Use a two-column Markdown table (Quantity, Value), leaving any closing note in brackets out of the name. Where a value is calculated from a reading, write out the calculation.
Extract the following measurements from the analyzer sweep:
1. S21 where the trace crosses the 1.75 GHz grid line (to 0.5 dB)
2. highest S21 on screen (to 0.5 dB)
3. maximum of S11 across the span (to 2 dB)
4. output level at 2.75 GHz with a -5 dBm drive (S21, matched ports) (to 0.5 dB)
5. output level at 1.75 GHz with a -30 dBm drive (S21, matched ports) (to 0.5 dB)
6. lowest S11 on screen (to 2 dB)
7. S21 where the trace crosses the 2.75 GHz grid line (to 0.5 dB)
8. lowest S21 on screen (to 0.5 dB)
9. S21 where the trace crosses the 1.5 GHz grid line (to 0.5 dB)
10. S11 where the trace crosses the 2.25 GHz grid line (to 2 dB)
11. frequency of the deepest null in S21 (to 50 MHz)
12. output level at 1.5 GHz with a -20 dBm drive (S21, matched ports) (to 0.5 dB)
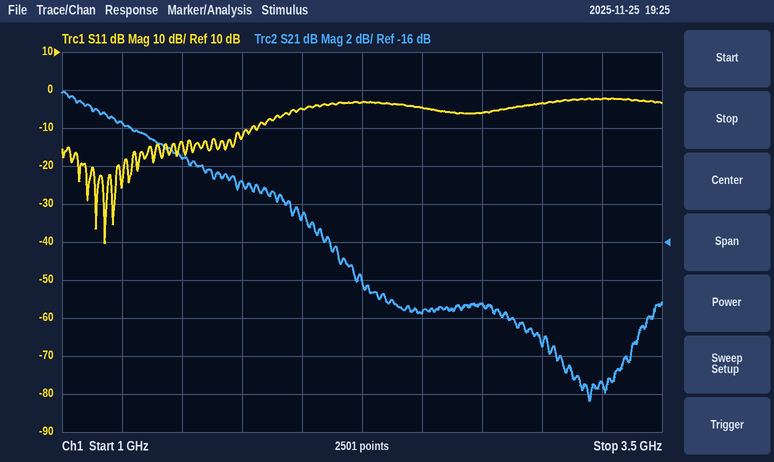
| Quantity | Value |
|---|---|
| S21 where the trace crosses the 1.75 GHz grid line | -13.0 dB |
| highest S21 on screen | -8.0 dB |
| maximum of S11 across the span | -2 dB |
| output level at 2.75 GHz with a -5 dBm drive (S21, matched ports) | -5 dBm + (-19.5 dB) = -24.5 dBm |
| output level at 1.75 GHz with a -30 dBm drive (S21, matched ports) | -30 dBm + (-13.0 dB) = -43.0 dBm |
| lowest S11 on screen | -40 dB |
| S21 where the trace crosses the 2.75 GHz grid line | -19.5 dB |
| lowest S21 on screen | -24.5 dB |
| S21 where the trace crosses the 1.5 GHz grid line | -11.5 dB |
| S11 where the trace crosses the 2.25 GHz grid line | -4 dB |
| frequency of the deepest null in S21 | 3.20 GHz |
| output level at 1.5 GHz with a -20 dBm drive (S21, matched ports) | -20 dBm + (-11.5 dB) = -31.5 dBm |
